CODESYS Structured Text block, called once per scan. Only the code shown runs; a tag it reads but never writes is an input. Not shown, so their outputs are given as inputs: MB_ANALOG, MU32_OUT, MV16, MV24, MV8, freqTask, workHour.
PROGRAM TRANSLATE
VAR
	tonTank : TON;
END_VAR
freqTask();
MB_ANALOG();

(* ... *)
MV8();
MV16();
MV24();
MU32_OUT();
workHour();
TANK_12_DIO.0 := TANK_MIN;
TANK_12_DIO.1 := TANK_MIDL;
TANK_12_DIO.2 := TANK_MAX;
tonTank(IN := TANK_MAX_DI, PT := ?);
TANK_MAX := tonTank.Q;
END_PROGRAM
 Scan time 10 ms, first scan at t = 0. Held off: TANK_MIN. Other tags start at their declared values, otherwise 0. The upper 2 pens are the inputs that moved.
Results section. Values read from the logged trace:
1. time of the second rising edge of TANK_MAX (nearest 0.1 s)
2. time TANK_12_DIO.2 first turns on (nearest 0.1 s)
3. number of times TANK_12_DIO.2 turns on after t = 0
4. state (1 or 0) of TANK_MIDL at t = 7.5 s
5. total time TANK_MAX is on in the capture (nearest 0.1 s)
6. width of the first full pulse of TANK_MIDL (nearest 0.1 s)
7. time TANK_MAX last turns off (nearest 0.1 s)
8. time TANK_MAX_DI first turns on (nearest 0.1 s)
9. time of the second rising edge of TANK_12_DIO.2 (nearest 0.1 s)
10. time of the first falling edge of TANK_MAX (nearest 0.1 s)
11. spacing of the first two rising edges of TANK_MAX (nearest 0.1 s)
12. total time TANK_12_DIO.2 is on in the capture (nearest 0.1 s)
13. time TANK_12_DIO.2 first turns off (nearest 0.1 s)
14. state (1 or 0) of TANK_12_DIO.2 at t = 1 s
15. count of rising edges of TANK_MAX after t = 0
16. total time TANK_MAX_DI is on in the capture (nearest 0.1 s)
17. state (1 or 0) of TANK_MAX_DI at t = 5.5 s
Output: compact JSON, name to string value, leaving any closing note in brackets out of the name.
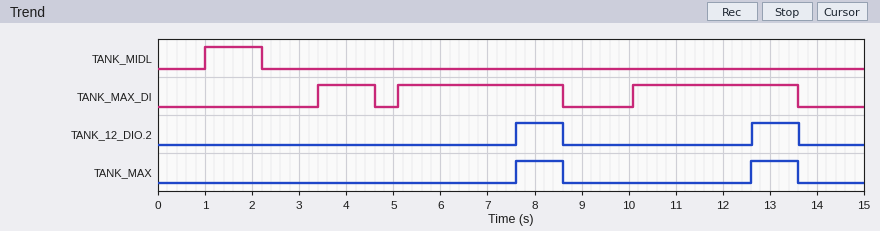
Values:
{"time of the second rising edge of TANK_MAX": "12.6 s", "time TANK_12_DIO.2 first turns on": "7.6 s", "number of times TANK_12_DIO.2 turns on after t = 0": "2", "state (1 or 0) of TANK_MIDL at t = 7.5 s": "0", "total time TANK_MAX is on in the capture": "2.0 s", "width of the first full pulse of TANK_MIDL": "1.2 s", "time TANK_MAX last turns off": "13.6 s", "time TANK_MAX_DI first turns on": "3.4 s", "time of the second rising edge of TANK_12_DIO.2": "12.6 s", "time of the first falling edge of TANK_MAX": "8.6 s", "spacing of the first two rising edges of TANK_MAX": "5.0 s", "total time TANK_12_DIO.2 is on in the capture": "2.0 s", "time TANK_12_DIO.2 first turns off": "8.6 s", "state (1 or 0) of TANK_12_DIO.2 at t = 1 s": "0", "count of rising edges of TANK_MAX after t = 0": "2", "total time TANK_MAX_DI is on in the capture": "8.2 s", "state (1 or 0) of TANK_MAX_DI at t = 5.5 s": "1"}
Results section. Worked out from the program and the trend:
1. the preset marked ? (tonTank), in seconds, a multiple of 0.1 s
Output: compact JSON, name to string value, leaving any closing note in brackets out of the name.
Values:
{"the preset marked ? (tonTank), in seconds, a multiple of 0.1 s": "2.5 s"}
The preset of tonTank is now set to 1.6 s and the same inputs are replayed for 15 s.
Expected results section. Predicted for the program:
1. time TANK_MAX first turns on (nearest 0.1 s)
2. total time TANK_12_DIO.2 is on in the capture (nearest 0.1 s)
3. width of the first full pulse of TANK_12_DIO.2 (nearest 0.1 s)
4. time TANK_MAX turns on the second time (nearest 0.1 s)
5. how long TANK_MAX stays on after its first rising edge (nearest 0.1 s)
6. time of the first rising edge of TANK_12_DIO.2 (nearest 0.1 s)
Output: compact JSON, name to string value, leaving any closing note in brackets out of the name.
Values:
{"time TANK_MAX first turns on": "6.7 s", "total time TANK_12_DIO.2 is on in the capture": "3.8 s", "width of the first full pulse of TANK_12_DIO.2": "1.9 s", "time TANK_MAX turns on the second time": "11.7 s", "how long TANK_MAX stays on after its first rising edge": "1.9 s", "time of the first rising edge of TANK_12_DIO.2": "6.7 s"}
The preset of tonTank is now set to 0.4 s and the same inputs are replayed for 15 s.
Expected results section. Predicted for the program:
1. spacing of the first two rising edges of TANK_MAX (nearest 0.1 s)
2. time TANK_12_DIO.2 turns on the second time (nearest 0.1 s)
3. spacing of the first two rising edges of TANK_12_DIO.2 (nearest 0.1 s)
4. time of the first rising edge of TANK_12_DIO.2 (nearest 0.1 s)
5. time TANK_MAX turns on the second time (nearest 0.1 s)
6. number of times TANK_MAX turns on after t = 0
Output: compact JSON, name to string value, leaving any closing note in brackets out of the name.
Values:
{"spacing of the first two rising edges of TANK_MAX": "1.7 s", "time TANK_12_DIO.2 turns on the second time": "5.5 s", "spacing of the first two rising edges of TANK_12_DIO.2": "1.7 s", "time of the first rising edge of TANK_12_DIO.2": "3.8 s", "time TANK_MAX turns on the second time": "5.5 s", "number of times TANK_MAX turns on after t = 0": "3"}
